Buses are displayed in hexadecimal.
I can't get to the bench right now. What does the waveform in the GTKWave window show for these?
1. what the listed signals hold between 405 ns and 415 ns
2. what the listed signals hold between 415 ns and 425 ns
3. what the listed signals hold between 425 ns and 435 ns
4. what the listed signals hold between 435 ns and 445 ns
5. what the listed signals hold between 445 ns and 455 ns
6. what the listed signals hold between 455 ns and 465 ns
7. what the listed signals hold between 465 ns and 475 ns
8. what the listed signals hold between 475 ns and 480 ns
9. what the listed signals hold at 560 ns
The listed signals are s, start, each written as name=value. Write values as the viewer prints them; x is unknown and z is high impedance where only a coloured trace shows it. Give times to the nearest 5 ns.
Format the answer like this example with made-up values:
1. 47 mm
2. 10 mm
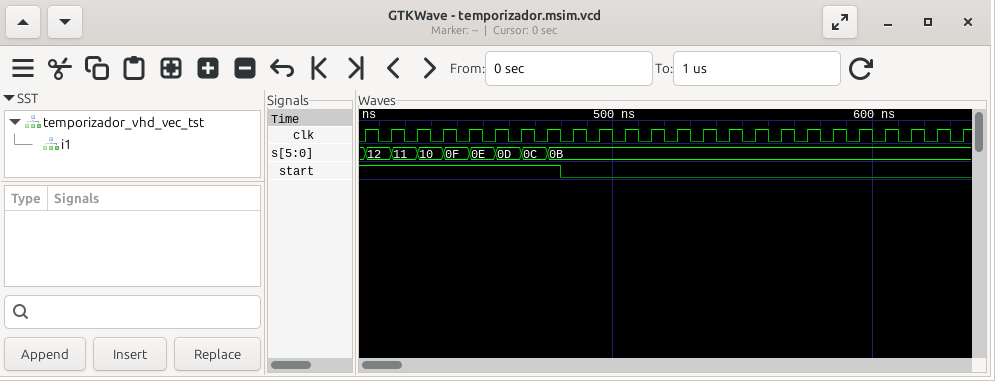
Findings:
1. s=12, start=1
2. s=11, start=1
3. s=10, start=1
4. s=0F, start=1
5. s=0E, start=1
6. s=0D, start=1
7. s=0C, start=1
8. s=0B, start=1
9. s=0B, start=0
